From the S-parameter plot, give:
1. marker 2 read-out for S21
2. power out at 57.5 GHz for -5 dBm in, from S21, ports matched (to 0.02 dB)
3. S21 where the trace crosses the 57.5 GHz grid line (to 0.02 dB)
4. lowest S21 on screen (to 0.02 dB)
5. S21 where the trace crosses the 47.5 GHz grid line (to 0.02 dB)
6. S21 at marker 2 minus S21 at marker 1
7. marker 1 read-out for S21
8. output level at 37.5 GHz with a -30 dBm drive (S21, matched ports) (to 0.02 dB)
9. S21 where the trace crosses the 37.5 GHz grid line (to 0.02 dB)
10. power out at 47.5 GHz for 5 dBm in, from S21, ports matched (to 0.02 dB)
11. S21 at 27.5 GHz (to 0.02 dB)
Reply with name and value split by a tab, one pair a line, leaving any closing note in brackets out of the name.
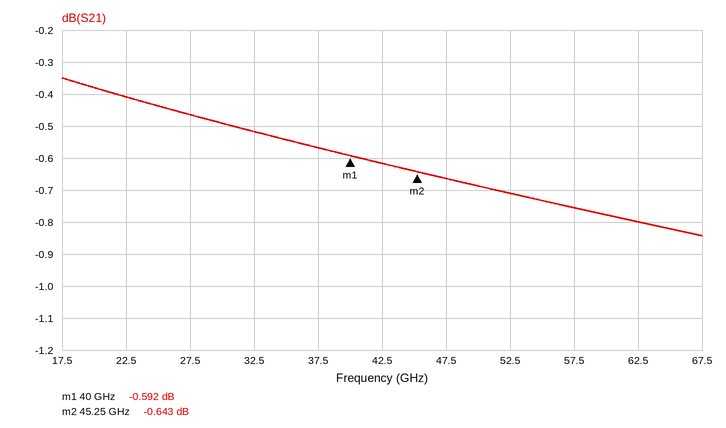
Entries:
marker 2 read-out for S21	-0.643 dB
power out at 57.5 GHz for -5 dBm in, from S21, ports matched	-5.76 dBm
S21 where the trace crosses the 57.5 GHz grid line	-0.76 dB
lowest S21 on screen	-0.84 dB
S21 where the trace crosses the 47.5 GHz grid line	-0.66 dB
S21 at marker 2 minus S21 at marker 1	-0.051 dB
marker 1 read-out for S21	-0.592 dB
output level at 37.5 GHz with a -30 dBm drive (S21, matched ports)	-30.56 dBm
S21 where the trace crosses the 37.5 GHz grid line	-0.56 dB
power out at 47.5 GHz for 5 dBm in, from S21, ports matched	4.34 dBm
S21 at 27.5 GHz	-0.46 dB
